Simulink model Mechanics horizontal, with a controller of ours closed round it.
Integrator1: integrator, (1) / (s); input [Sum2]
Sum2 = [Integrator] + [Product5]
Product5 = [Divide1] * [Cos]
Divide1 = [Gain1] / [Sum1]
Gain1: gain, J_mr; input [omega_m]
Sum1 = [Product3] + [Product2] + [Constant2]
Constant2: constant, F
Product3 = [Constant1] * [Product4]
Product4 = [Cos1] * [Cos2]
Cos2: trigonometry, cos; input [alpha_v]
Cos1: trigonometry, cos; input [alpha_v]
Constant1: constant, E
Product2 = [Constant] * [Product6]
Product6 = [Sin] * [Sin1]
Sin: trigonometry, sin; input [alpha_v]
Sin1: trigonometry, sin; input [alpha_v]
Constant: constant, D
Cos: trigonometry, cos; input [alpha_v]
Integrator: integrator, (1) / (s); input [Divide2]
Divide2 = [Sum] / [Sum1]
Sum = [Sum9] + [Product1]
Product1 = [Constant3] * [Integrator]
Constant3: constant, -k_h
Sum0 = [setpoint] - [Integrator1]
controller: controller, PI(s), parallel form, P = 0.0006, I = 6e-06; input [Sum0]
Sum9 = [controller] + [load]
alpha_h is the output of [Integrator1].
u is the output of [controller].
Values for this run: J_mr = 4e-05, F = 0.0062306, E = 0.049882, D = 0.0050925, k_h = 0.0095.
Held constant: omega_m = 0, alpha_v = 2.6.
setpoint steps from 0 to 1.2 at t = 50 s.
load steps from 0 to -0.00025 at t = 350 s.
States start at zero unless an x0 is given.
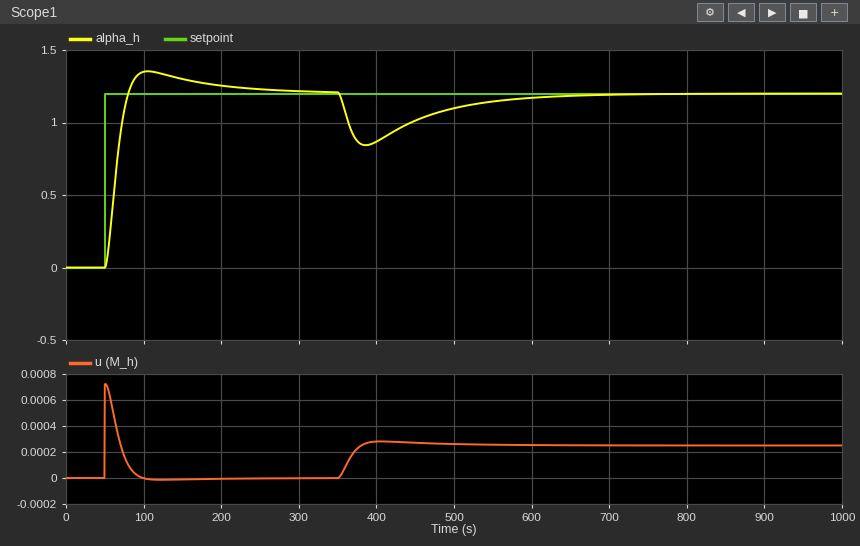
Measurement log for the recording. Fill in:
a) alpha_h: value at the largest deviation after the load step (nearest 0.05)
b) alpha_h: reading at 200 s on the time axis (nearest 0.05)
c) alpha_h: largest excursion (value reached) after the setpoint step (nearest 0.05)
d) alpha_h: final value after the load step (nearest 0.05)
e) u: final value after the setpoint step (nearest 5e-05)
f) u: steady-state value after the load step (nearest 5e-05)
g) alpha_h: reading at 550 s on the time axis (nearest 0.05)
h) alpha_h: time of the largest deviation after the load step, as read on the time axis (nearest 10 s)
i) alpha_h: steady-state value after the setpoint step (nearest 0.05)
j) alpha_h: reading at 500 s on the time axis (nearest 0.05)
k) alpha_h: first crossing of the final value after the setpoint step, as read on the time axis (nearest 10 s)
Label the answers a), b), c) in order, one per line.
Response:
a) 0.85
b) 1.25
c) 1.35
d) 1.20
e) 0.00000
f) 0.00025
g) 1.15
h) 390 s
i) 1.20
j) 1.10
k) 80 s
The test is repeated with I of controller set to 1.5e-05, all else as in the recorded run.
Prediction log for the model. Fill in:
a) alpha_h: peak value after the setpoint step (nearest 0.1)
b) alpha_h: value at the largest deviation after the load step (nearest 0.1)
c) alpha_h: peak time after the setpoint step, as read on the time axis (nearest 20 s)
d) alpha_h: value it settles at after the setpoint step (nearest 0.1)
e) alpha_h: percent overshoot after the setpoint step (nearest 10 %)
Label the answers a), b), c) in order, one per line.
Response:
a) 1.5
b) 0.9
c) 100 s
d) 1.2
e) 30 %
